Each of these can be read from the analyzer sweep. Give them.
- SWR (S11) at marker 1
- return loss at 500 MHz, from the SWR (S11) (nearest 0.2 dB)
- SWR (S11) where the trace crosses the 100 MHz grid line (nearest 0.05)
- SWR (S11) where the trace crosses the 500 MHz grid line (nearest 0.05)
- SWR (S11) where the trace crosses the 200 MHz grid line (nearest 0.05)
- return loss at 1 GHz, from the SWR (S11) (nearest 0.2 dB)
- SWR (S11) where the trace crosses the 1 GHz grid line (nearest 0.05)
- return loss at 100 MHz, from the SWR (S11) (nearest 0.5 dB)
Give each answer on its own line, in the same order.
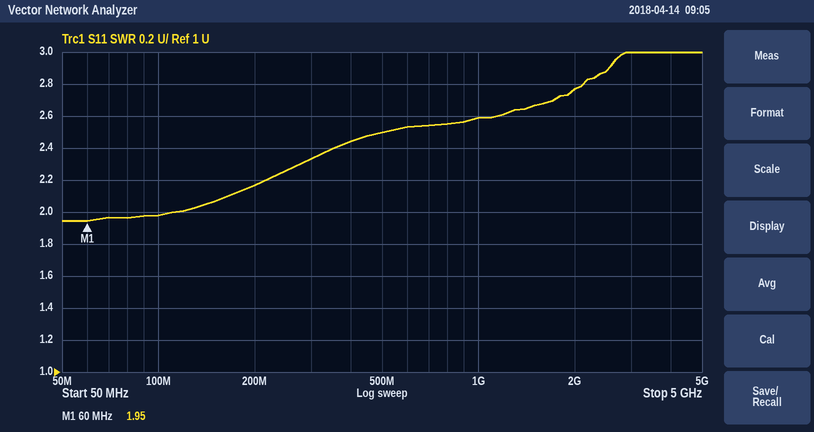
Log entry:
1.95
7.4 dB
2.00
2.50
2.15
7.0 dB
2.60
9.5 dB
